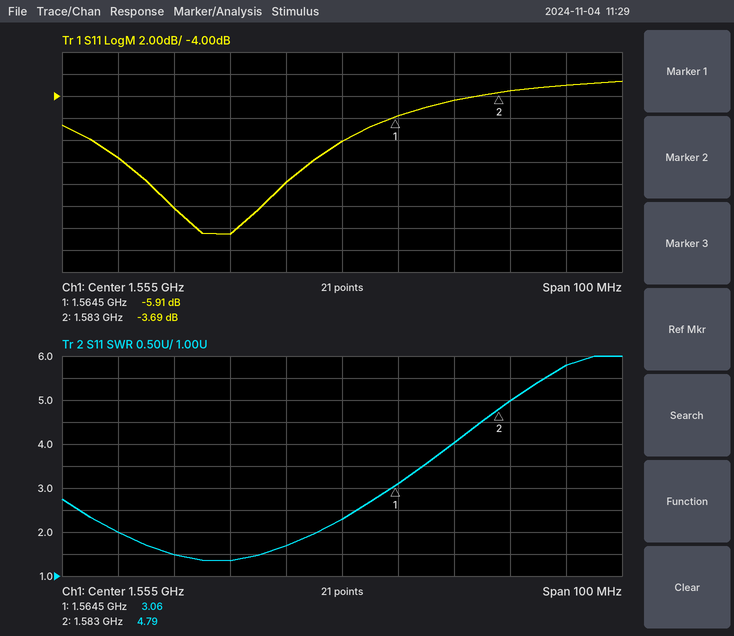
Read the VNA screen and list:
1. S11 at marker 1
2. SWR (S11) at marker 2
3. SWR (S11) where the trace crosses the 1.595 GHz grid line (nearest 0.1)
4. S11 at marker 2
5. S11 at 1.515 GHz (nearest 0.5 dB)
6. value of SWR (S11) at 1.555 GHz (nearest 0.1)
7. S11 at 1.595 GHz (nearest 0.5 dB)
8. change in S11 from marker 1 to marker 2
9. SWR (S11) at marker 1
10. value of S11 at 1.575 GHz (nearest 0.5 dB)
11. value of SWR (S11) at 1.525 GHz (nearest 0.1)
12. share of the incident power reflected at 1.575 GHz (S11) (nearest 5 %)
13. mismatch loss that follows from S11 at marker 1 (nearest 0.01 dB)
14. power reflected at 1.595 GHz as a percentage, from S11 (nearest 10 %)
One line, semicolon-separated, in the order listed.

-5.91 dB; 4.79; 5.8; -3.69 dB; -9.5 dB; 2.3; -3.0 dB; 2.22 dB; 3.06; -4.5 dB; 1.5; 35 %; 1.29 dB; 50 %
